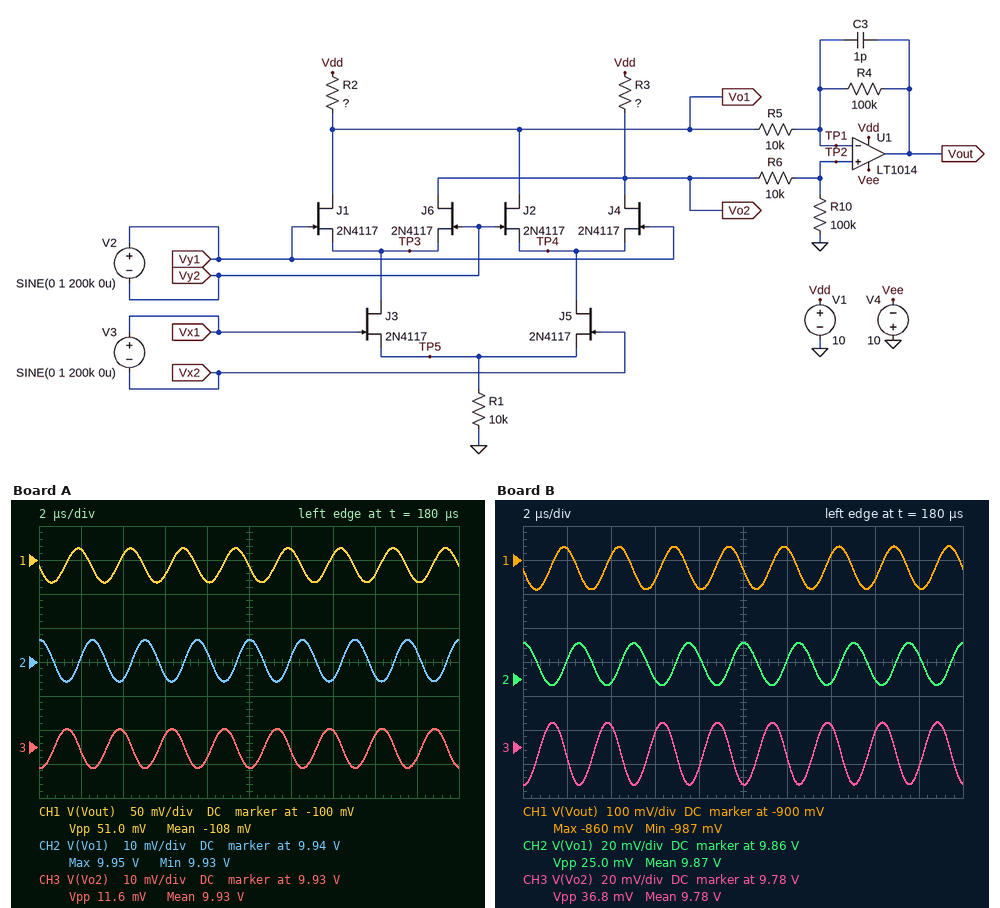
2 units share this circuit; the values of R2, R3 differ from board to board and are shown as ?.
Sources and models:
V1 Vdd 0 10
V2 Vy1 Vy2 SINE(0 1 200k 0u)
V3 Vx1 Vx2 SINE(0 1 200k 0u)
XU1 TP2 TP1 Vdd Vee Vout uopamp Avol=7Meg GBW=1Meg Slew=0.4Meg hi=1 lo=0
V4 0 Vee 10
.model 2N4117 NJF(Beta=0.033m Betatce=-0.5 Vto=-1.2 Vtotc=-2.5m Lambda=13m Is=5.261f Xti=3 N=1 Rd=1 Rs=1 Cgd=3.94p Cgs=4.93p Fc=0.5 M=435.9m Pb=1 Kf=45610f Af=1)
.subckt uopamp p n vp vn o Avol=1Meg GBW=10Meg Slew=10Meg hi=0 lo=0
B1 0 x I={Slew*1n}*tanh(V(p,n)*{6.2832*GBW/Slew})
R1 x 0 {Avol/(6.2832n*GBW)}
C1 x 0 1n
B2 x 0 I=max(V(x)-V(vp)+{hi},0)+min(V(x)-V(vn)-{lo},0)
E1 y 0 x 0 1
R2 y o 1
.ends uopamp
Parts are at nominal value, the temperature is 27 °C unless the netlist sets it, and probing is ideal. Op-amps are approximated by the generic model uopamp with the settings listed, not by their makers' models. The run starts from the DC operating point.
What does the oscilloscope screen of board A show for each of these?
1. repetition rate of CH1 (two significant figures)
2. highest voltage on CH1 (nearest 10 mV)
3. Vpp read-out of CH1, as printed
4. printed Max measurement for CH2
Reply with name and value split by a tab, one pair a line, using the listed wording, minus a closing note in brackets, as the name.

repetition rate of CH1	400 kHz
highest voltage on CH1	-80 mV
Vpp read-out of CH1, as printed	51.0 mV
printed Max measurement for CH2	9.95 V
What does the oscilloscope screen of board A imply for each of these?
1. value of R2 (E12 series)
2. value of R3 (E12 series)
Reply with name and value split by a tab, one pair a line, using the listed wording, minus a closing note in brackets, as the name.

value of R2	390 Ω
value of R3	560 Ω
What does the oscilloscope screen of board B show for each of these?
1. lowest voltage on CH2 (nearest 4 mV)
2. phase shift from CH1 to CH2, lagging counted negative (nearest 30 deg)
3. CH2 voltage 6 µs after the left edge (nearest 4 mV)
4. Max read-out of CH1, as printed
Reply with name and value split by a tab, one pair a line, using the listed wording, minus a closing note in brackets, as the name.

lowest voltage on CH2	9.856 V
phase shift from CH1 to CH2, lagging counted negative	-90 deg
CH2 voltage 6 µs after the left edge	9.860 V
Max read-out of CH1, as printed	-860 mV
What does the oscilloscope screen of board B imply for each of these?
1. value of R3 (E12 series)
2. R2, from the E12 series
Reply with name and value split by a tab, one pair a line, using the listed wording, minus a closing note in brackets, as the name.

value of R3	1.8 kΩ
R2, from the E12 series	820 Ω
